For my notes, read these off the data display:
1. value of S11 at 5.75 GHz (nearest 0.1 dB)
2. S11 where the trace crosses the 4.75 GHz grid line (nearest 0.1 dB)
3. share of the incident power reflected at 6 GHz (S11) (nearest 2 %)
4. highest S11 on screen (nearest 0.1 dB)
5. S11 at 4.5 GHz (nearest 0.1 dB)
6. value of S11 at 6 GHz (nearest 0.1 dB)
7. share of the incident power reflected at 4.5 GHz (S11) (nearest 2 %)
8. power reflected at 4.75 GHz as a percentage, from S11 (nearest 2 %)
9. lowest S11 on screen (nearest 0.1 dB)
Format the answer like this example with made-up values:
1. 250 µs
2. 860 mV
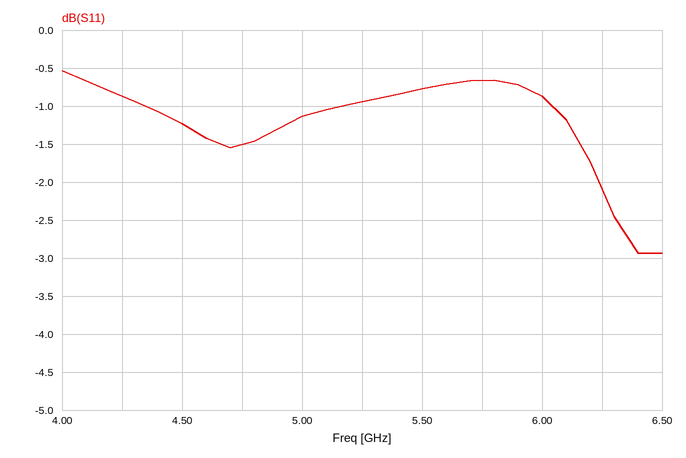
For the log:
1. -0.7 dB
2. -1.5 dB
3. 82 %
4. -0.5 dB
5. -1.2 dB
6. -0.9 dB
7. 76 %
8. 70 %
9. -2.9 dB
